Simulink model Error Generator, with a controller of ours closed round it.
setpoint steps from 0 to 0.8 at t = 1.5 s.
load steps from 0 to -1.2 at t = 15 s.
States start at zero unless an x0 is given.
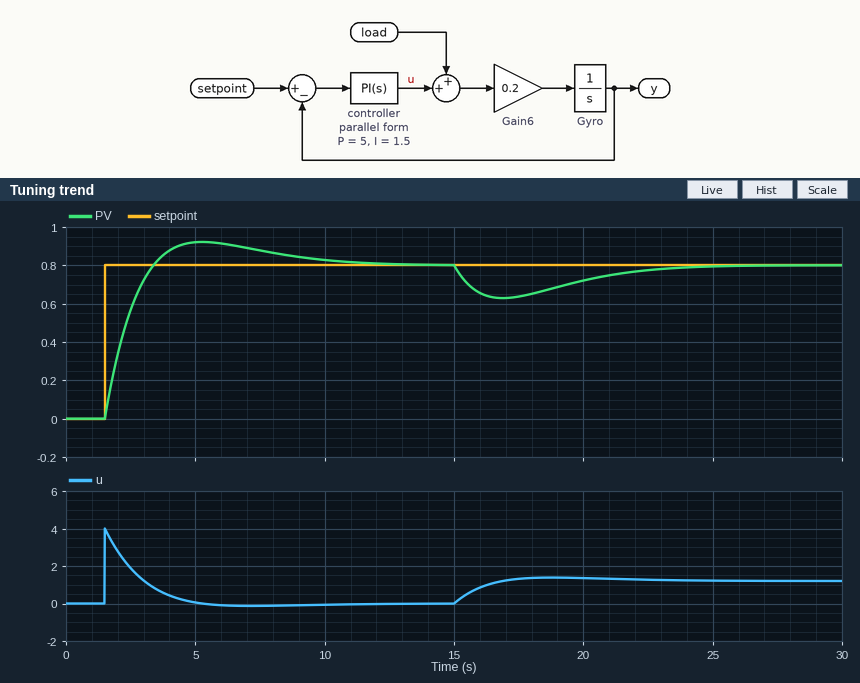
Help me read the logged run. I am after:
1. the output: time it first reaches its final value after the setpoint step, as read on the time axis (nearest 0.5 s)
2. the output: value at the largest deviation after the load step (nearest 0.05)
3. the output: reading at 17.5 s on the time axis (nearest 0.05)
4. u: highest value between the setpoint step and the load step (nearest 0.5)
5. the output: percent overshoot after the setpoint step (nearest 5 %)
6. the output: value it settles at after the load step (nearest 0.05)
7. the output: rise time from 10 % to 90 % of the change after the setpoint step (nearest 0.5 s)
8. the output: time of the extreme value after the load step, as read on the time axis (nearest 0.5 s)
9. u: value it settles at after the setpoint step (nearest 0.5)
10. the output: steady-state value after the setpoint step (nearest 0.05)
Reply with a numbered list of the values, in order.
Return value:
1. 3.5 s
2. 0.65
3. 0.65
4. 4.0
5. 15 %
6. 0.80
7. 1.5 s
8. 17.0 s
9. 0.0
10. 0.80
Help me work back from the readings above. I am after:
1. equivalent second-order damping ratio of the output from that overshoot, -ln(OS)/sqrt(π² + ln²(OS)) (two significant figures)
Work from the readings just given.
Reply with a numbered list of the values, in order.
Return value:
1. 0.52
